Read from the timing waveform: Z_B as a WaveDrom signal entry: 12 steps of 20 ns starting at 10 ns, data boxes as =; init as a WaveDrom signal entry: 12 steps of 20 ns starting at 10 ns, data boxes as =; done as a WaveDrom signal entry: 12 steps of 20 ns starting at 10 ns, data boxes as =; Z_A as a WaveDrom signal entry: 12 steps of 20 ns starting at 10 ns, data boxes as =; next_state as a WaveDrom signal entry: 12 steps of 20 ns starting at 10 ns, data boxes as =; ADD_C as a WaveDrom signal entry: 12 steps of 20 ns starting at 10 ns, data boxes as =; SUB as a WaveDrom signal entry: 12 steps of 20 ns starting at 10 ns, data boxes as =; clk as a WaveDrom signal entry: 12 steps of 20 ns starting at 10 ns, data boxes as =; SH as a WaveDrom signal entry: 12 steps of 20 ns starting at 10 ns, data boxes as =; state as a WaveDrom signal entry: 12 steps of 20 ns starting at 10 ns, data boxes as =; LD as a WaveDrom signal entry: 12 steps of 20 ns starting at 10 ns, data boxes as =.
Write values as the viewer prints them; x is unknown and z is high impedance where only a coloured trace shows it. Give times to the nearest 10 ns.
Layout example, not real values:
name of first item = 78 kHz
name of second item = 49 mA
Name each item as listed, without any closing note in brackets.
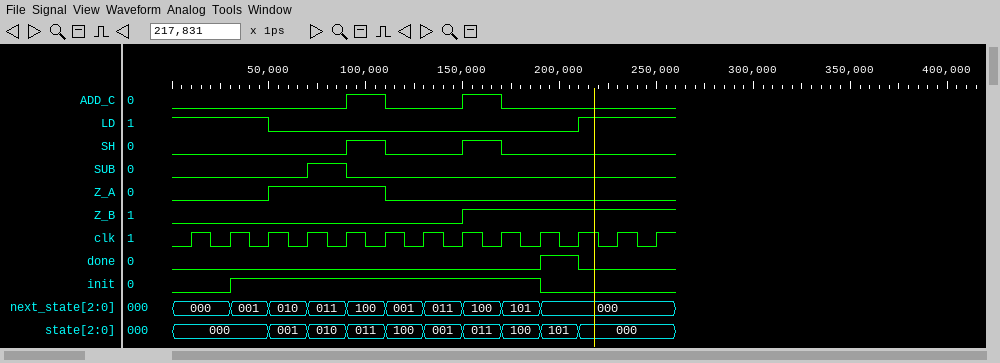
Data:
Z_B as a WaveDrom signal entry: 12 steps of 20 ns starting at 10 ns, data boxes as = = {name: 'Z_B', wave: '0......1....'}
init as a WaveDrom signal entry: 12 steps of 20 ns starting at 10 ns, data boxes as = = {name: 'init', wave: '01.......0..'}
done as a WaveDrom signal entry: 12 steps of 20 ns starting at 10 ns, data boxes as = = {name: 'done', wave: '0........10.'}
Z_A as a WaveDrom signal entry: 12 steps of 20 ns starting at 10 ns, data boxes as = = {name: 'Z_A', wave: '0.1..0......'}
next_state as a WaveDrom signal entry: 12 steps of 20 ns starting at 10 ns, data boxes as = = {name: 'next_state', wave: '==========..', data: '000 001 010 011 100 001 011 100 101 000'}
ADD_C as a WaveDrom signal entry: 12 steps of 20 ns starting at 10 ns, data boxes as = = {name: 'ADD_C', wave: '0...10.10...'}
SUB as a WaveDrom signal entry: 12 steps of 20 ns starting at 10 ns, data boxes as = = {name: 'SUB', wave: '0..10.......'}
clk as a WaveDrom signal entry: 12 steps of 20 ns starting at 10 ns, data boxes as = = {name: 'clk', wave: 'p...........'}
SH as a WaveDrom signal entry: 12 steps of 20 ns starting at 10 ns, data boxes as = = {name: 'SH', wave: '0...10.10...'}
state as a WaveDrom signal entry: 12 steps of 20 ns starting at 10 ns, data boxes as = = {name: 'state', wave: '=.=========.', data: '000 001 010 011 100 001 011 100 101 000'}
LD as a WaveDrom signal entry: 12 steps of 20 ns starting at 10 ns, data boxes as = = {name: 'LD', wave: '1.0.......1.'}
